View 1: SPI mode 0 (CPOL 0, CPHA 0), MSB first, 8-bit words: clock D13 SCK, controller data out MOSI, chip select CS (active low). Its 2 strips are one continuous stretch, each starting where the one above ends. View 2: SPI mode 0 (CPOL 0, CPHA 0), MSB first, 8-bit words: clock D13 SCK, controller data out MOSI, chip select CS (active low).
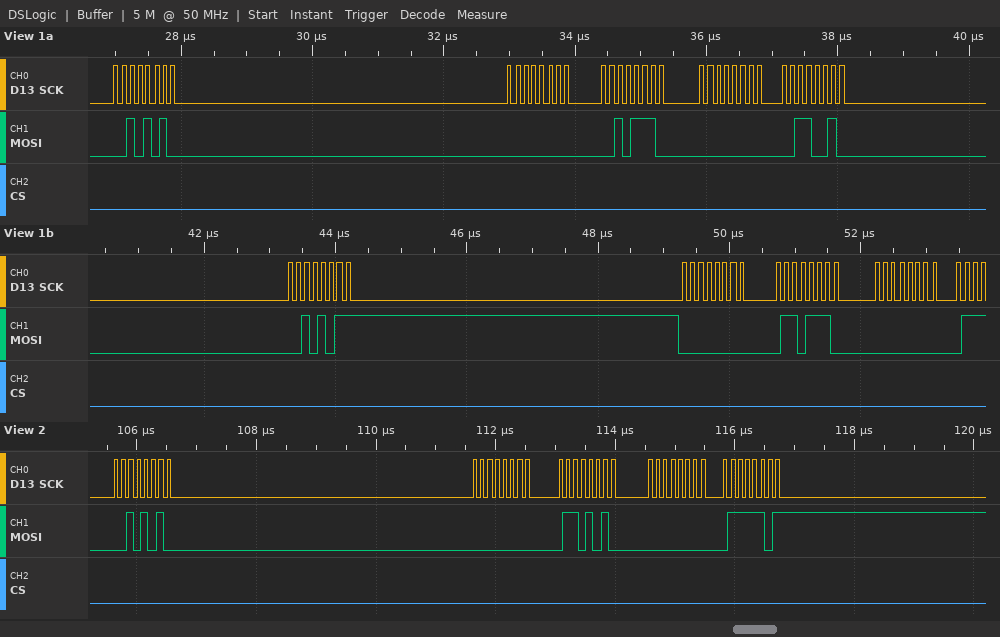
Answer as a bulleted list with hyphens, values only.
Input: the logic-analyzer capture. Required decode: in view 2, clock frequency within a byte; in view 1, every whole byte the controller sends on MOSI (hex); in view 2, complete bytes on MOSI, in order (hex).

- 8 MHz
- 2A 00 2E 00 32 2B 00 6E 00
- 2A 00 6A 00 7D
